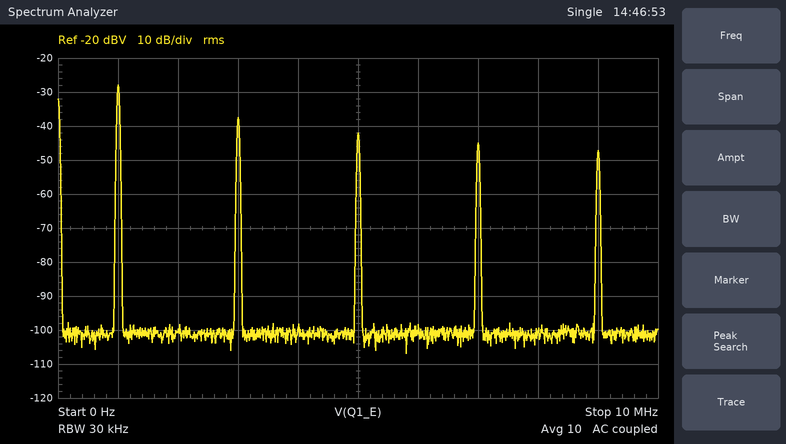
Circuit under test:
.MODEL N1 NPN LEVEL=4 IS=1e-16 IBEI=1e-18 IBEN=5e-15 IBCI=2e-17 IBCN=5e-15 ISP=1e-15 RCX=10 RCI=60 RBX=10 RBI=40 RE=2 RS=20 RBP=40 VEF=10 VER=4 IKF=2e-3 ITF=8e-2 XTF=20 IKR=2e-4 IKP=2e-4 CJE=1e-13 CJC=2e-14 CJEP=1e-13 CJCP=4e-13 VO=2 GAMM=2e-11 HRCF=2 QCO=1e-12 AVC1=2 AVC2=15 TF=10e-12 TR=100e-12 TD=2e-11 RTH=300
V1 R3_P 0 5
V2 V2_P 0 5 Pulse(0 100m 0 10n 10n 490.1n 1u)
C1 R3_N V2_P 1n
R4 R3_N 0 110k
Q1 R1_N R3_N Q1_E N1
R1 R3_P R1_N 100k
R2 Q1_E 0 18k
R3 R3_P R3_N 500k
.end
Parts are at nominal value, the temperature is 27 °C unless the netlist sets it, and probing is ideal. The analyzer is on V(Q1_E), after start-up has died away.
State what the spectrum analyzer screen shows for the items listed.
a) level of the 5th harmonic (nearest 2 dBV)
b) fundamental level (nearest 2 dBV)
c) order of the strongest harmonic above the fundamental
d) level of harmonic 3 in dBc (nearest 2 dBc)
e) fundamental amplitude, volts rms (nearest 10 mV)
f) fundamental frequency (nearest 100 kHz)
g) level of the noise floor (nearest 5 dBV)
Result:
-42 dBV
-28 dBV
3
-10 dBc
40 mV
1.0 MHz
-100 dBV
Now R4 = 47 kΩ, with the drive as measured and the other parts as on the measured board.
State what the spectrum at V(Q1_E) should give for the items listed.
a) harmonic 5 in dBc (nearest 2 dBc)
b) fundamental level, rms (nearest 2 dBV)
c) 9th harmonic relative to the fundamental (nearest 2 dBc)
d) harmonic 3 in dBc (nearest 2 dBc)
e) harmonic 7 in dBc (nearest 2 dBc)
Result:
0 dBc
-64 dBV
0 dBc
0 dBc
0 dBc
